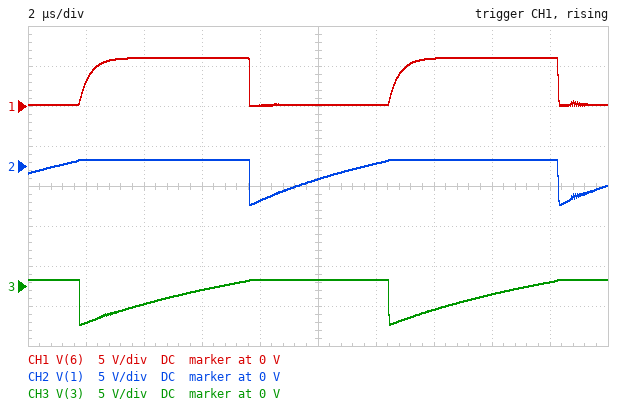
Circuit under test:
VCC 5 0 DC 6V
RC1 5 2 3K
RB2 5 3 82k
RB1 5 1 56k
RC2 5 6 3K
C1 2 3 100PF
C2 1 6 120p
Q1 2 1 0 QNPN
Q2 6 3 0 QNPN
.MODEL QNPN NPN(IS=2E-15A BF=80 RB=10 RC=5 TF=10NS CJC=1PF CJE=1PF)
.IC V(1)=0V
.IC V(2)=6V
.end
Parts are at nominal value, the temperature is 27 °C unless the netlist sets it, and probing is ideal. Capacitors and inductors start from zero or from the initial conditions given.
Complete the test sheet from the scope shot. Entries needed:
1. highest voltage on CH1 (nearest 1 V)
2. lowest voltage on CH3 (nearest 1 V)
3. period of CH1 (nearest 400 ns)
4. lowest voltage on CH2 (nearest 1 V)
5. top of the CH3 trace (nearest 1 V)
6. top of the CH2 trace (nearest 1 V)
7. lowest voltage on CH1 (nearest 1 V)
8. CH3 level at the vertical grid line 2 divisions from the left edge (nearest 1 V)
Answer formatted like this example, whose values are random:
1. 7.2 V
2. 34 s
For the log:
1. 6 V
2. -5 V
3. 10.8 µs
4. -5 V
5. 1 V
6. 1 V
7. 0 V
8. -2 V
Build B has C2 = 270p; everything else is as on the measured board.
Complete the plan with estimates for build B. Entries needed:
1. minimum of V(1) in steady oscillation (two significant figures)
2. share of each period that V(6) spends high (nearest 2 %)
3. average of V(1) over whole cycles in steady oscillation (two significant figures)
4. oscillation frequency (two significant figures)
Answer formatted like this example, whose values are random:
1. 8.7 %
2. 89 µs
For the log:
1. -5.1 V
2. 32 %
3. -960 mV
4. 60 kHz
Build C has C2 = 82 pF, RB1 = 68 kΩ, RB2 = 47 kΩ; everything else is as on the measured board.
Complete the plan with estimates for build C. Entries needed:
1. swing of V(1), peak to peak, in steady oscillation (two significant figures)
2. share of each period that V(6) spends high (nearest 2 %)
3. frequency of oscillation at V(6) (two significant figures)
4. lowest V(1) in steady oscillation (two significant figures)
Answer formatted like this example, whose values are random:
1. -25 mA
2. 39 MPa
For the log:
1. 5.6 V
2. 44 %
3. 140 kHz
4. -4.8 V
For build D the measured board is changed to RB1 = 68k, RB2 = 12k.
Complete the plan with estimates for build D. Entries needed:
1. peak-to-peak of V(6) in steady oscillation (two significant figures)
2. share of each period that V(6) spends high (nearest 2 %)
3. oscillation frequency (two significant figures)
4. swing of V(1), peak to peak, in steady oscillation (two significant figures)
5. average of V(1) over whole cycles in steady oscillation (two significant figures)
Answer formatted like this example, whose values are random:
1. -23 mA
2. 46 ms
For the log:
1. 5.4 V
2. 10 %
3. 160 kHz
4. 5.1 V
5. -1.2 V
